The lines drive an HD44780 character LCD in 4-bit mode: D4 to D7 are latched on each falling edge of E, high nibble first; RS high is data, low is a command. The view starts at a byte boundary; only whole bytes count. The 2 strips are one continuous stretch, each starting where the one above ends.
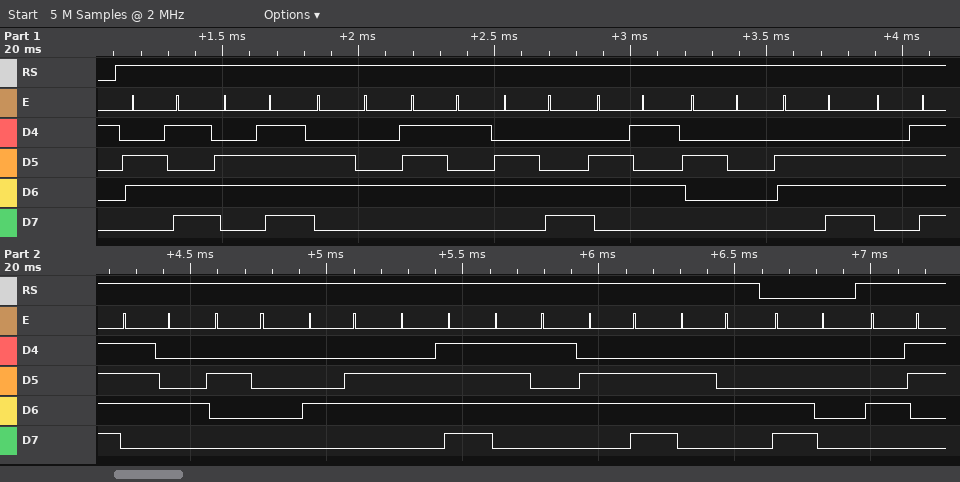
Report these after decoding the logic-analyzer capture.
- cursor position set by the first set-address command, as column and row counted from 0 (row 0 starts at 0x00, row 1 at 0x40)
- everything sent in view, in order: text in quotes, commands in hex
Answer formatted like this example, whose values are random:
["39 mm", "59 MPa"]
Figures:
["column 0, row 1", "\"module not Found\" 0xC0 \"C\""]
